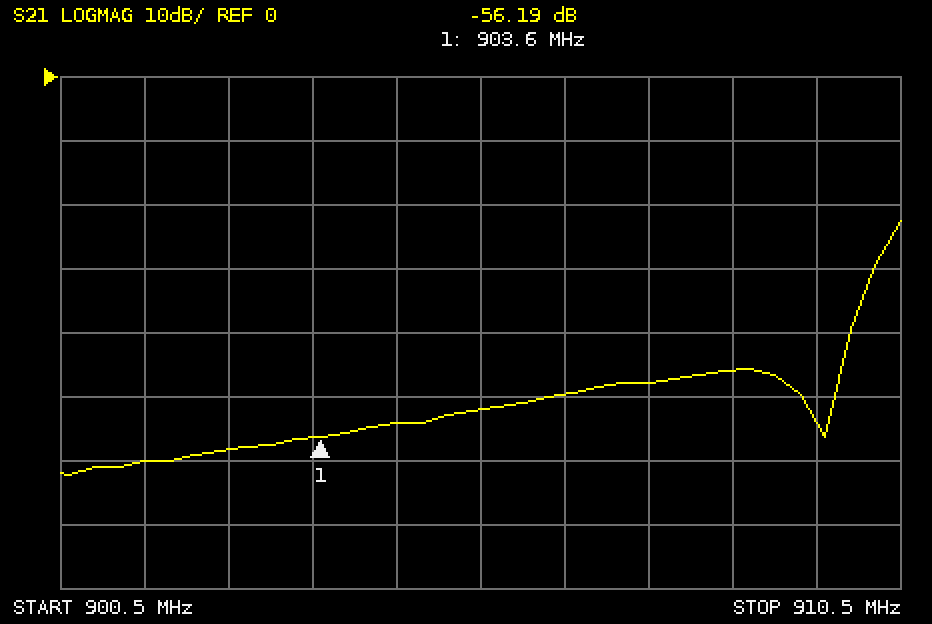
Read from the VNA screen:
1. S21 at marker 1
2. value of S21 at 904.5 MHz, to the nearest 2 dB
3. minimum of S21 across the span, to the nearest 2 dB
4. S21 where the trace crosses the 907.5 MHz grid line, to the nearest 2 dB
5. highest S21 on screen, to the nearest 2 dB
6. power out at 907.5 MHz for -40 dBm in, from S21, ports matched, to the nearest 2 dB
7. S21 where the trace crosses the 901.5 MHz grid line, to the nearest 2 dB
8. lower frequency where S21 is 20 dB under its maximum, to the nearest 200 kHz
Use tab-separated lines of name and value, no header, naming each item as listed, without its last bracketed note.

S21 at marker 1	-56.19 dB
value of S21 at 904.5 MHz, to the nearest 2 dB	-54 dB
minimum of S21 across the span, to the nearest 2 dB	-62 dB
S21 where the trace crosses the 907.5 MHz grid line, to the nearest 2 dB	-48 dB
highest S21 on screen, to the nearest 2 dB	-22 dB
power out at 907.5 MHz for -40 dBm in, from S21, ports matched, to the nearest 2 dB	-88 dBm
S21 where the trace crosses the 901.5 MHz grid line, to the nearest 2 dB	-60 dB
lower frequency where S21 is 20 dB under its maximum, to the nearest 200 kHz	909.8 MHz
